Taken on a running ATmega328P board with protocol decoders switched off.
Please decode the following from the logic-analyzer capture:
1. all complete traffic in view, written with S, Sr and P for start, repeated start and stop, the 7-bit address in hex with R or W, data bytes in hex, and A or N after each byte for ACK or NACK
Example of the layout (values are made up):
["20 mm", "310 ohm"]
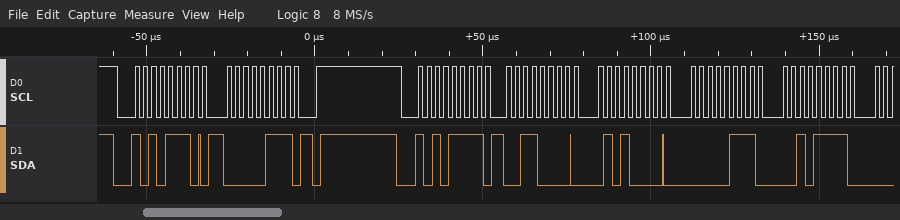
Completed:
["S 57W A 07 A P S 57R A 30 A 50 A 07 A 2F A"]
